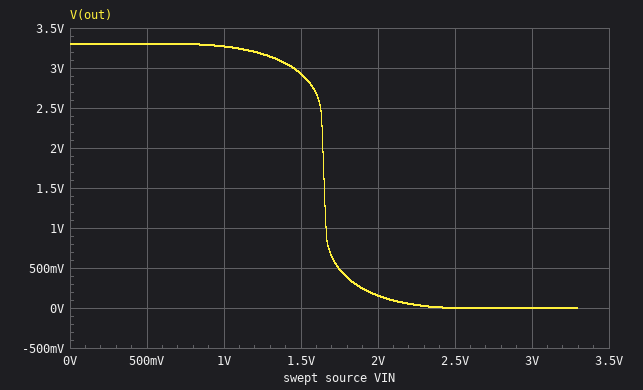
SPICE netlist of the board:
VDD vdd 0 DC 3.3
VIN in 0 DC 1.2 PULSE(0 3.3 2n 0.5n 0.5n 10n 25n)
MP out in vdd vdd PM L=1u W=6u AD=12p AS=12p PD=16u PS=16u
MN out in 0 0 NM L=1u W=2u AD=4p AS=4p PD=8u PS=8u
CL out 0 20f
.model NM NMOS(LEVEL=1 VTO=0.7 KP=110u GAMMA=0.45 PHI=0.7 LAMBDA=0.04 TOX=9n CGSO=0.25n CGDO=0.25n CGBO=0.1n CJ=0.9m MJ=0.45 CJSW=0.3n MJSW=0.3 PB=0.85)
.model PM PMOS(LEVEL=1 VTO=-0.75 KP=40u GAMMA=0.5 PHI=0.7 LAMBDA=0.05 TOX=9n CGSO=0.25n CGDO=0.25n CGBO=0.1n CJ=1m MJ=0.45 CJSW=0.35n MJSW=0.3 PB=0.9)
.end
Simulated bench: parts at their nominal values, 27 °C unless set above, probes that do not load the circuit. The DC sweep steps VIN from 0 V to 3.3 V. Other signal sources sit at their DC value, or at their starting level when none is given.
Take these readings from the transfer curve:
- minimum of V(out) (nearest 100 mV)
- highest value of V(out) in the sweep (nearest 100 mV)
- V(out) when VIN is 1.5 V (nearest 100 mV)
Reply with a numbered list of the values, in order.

1. 0 V
2. 3.3 V
3. 2.9 V
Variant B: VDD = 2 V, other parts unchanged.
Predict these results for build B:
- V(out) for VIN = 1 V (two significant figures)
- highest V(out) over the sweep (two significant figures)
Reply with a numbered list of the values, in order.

1. 170 mV
2. 2.0 V
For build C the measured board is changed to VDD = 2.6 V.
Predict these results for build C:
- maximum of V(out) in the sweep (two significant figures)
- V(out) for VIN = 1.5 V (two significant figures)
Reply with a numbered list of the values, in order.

1. 2.6 V
2. 100 mV
